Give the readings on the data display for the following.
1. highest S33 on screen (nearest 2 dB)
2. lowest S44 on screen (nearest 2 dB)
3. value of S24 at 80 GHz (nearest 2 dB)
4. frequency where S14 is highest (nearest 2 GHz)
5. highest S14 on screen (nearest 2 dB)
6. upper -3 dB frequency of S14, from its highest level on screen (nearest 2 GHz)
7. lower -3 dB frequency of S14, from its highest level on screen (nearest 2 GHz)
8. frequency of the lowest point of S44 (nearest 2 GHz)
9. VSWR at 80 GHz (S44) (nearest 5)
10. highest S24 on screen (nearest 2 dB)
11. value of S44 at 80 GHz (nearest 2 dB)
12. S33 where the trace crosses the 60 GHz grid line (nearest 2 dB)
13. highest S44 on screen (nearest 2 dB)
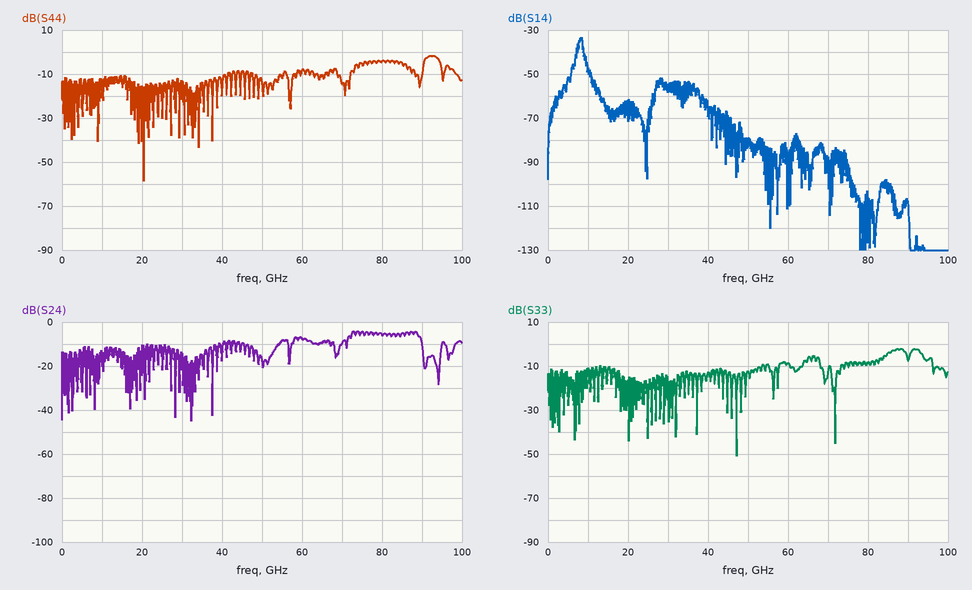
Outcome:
-2 dB
-58 dB
-6 dB
8 GHz
-34 dB
8 GHz
8 GHz
20 GHz
5
-4 dB
-4 dB
-8 dB
-2 dB
